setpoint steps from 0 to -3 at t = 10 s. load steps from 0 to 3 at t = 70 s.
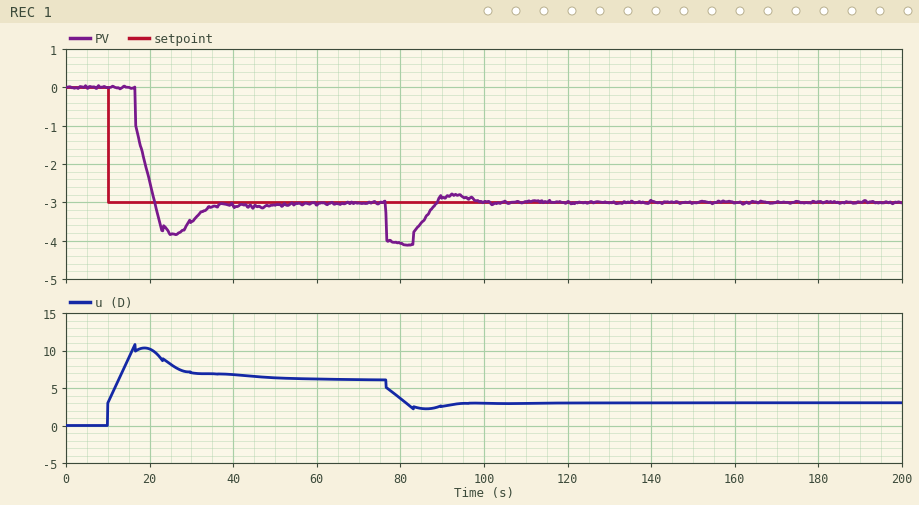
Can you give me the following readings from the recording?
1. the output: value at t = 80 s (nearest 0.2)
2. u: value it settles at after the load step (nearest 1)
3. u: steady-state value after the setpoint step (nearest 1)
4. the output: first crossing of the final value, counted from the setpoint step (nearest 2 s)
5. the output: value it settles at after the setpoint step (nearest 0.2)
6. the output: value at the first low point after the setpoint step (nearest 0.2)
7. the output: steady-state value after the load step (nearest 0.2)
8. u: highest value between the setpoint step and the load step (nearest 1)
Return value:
-4.0
3
6
12 s
-3.0
-3.8
-3.0
11
